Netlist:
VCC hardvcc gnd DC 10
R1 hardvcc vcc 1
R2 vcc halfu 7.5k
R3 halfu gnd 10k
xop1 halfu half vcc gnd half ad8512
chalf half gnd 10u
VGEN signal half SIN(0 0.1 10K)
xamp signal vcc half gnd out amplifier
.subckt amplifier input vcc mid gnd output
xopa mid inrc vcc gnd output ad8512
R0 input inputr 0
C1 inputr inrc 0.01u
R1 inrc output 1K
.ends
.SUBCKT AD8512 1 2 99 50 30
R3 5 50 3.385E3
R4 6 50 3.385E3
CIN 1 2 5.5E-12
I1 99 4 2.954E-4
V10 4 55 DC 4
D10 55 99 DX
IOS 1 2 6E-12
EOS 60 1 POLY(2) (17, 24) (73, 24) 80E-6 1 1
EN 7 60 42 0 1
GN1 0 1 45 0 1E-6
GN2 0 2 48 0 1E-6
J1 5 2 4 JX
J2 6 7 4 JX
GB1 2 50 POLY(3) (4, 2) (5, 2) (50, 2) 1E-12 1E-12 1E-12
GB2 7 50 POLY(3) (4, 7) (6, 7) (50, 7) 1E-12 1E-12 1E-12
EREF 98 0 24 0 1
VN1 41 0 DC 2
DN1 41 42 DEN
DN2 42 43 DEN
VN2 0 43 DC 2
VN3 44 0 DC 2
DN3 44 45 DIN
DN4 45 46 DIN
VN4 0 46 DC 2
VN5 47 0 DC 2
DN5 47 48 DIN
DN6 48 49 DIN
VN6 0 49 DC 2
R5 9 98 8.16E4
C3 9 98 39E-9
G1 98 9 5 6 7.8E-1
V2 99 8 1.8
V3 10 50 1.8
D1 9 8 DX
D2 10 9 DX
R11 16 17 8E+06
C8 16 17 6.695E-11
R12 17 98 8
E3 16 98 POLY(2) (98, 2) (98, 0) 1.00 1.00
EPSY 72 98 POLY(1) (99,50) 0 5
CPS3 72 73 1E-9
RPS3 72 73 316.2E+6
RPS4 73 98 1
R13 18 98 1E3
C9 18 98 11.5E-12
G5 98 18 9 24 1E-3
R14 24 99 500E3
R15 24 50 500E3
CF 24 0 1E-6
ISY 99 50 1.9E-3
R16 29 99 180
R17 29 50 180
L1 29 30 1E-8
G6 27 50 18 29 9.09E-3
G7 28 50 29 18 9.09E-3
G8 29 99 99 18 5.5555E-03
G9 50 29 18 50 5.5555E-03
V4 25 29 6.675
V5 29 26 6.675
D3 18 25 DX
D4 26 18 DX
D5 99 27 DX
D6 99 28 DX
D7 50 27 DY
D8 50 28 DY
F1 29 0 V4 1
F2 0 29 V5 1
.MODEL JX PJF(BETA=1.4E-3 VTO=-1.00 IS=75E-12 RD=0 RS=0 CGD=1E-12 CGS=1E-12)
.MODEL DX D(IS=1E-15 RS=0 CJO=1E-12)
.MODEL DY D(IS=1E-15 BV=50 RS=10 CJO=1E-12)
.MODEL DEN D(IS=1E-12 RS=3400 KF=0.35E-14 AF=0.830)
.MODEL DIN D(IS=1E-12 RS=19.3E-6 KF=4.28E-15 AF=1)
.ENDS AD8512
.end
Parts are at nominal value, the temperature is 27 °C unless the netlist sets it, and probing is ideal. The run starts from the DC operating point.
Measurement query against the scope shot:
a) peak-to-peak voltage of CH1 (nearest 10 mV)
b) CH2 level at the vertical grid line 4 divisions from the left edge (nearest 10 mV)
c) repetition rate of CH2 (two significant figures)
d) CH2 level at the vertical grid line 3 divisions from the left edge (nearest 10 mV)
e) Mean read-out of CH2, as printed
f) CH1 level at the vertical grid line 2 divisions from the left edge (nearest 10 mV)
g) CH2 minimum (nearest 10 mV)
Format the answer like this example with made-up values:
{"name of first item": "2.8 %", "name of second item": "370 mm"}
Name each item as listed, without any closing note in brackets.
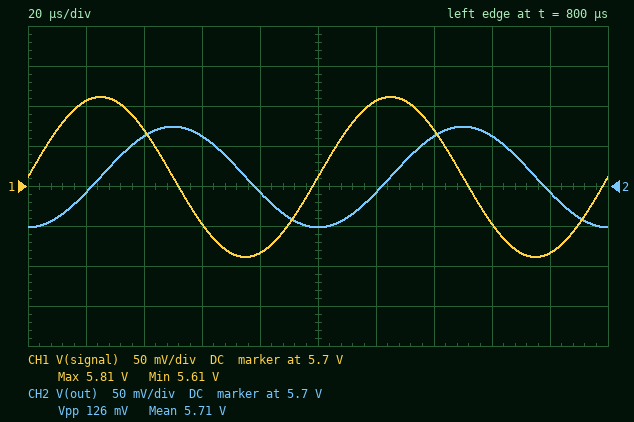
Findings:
{"peak-to-peak voltage of CH1": "200 mV", "CH2 level at the vertical grid line 4 divisions from the left edge": "5.69 V", "repetition rate of CH2": "10 kHz", "CH2 level at the vertical grid line 3 divisions from the left edge": "5.76 V", "Mean read-out of CH2, as printed": "5.71 V", "CH1 level at the vertical grid line 2 divisions from the left edge": "5.77 V", "CH2 minimum": "5.65 V"}
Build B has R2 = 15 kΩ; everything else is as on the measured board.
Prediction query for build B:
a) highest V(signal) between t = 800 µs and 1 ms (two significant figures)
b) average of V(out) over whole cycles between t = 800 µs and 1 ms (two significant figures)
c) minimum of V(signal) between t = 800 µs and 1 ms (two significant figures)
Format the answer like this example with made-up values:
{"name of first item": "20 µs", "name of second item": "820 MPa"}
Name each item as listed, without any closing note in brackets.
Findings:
{"highest V(signal) between t = 800 µs and 1 ms": "4.1 V", "average of V(out) over whole cycles between t = 800 µs and 1 ms": "4.0 V", "minimum of V(signal) between t = 800 µs and 1 ms": "3.9 V"}
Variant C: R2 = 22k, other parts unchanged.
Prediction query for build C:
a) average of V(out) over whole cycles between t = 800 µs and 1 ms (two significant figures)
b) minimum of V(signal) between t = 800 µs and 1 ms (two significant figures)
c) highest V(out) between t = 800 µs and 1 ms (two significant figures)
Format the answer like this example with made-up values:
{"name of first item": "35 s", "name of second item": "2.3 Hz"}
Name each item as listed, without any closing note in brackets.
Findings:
{"average of V(out) over whole cycles between t = 800 µs and 1 ms": "3.1 V", "minimum of V(signal) between t = 800 µs and 1 ms": "3.0 V", "highest V(out) between t = 800 µs and 1 ms": "3.2 V"}
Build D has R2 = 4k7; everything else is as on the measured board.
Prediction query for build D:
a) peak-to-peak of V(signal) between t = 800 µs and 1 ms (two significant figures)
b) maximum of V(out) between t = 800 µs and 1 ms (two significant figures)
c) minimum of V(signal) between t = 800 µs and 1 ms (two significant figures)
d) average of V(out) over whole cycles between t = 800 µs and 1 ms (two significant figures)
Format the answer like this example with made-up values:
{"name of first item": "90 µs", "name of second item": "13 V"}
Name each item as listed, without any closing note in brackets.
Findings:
{"peak-to-peak of V(signal) between t = 800 µs and 1 ms": "200 mV", "maximum of V(out) between t = 800 µs and 1 ms": "6.9 V", "minimum of V(signal) between t = 800 µs and 1 ms": "6.7 V", "average of V(out) over whole cycles between t = 800 µs and 1 ms": "6.8 V"}
